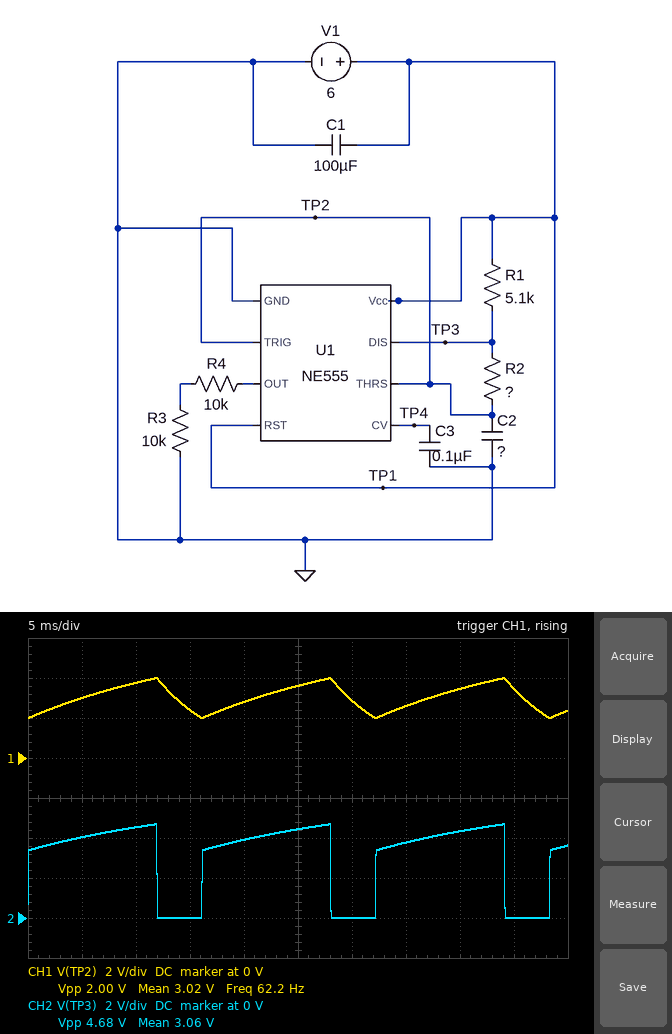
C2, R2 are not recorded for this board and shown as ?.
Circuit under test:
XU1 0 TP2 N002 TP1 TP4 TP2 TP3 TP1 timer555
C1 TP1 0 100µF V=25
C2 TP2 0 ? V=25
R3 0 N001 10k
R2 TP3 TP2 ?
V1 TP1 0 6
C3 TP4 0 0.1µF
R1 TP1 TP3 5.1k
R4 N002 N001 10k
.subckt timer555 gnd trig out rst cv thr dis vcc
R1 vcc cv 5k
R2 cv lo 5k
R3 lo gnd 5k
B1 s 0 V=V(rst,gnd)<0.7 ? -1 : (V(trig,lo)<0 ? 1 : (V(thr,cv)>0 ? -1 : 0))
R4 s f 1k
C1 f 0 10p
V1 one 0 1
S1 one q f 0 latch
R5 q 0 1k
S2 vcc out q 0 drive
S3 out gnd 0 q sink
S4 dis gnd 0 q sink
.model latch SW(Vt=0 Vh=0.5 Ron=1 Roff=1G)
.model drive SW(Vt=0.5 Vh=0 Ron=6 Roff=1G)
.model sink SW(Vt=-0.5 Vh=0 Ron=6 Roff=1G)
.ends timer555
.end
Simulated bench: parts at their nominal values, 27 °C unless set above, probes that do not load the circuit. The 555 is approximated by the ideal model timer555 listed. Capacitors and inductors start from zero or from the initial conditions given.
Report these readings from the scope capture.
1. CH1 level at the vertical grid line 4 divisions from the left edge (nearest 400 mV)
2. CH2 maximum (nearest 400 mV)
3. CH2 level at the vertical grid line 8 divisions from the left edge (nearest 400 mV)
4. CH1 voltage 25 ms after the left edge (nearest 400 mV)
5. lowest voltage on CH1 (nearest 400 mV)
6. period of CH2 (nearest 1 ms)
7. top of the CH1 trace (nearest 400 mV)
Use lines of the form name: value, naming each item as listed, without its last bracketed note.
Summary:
CH1 level at the vertical grid line 4 divisions from the left edge: 2.8 V
CH2 maximum: 4.8 V
CH2 level at the vertical grid line 8 divisions from the left edge: 4.4 V
CH1 voltage 25 ms after the left edge: 3.6 V
lowest voltage on CH1: 2.0 V
period of CH2: 16 ms
top of the CH1 trace: 4.0 V
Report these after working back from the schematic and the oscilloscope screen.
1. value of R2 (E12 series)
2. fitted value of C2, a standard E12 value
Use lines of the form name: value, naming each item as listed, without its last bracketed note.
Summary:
value of R2: 2.7 kΩ
fitted value of C2, a standard E12 value: 2.2 µF
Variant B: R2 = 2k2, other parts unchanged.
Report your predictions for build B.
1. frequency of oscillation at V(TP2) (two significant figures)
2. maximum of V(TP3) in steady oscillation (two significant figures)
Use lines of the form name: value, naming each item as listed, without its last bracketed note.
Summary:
frequency of oscillation at V(TP2): 69 Hz
maximum of V(TP3) in steady oscillation: 4.6 V
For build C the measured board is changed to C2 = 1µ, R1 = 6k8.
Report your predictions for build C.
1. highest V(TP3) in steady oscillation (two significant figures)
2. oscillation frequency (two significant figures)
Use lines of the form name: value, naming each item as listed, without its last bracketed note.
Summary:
highest V(TP3) in steady oscillation: 4.6 V
oscillation frequency: 120 Hz
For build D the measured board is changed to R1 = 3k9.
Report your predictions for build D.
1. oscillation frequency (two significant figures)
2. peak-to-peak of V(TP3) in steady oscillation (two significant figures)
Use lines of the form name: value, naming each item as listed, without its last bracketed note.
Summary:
oscillation frequency: 70 Hz
peak-to-peak of V(TP3) in steady oscillation: 4.8 V
